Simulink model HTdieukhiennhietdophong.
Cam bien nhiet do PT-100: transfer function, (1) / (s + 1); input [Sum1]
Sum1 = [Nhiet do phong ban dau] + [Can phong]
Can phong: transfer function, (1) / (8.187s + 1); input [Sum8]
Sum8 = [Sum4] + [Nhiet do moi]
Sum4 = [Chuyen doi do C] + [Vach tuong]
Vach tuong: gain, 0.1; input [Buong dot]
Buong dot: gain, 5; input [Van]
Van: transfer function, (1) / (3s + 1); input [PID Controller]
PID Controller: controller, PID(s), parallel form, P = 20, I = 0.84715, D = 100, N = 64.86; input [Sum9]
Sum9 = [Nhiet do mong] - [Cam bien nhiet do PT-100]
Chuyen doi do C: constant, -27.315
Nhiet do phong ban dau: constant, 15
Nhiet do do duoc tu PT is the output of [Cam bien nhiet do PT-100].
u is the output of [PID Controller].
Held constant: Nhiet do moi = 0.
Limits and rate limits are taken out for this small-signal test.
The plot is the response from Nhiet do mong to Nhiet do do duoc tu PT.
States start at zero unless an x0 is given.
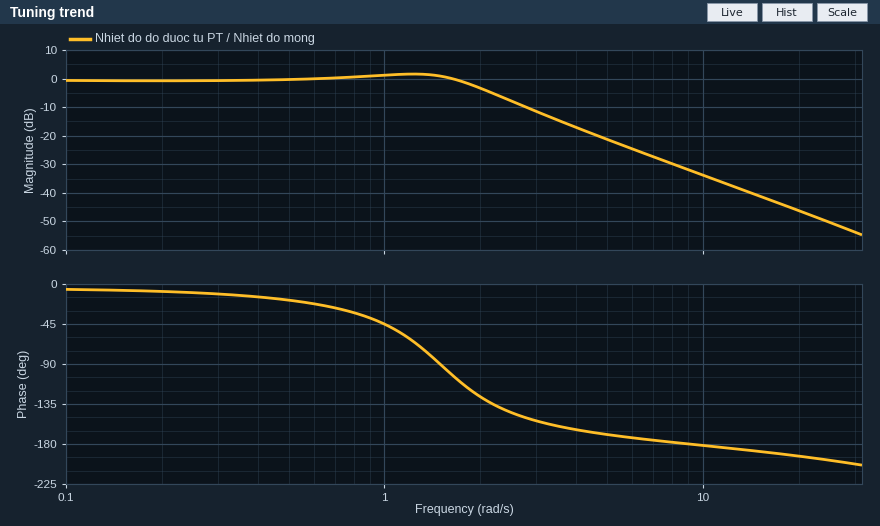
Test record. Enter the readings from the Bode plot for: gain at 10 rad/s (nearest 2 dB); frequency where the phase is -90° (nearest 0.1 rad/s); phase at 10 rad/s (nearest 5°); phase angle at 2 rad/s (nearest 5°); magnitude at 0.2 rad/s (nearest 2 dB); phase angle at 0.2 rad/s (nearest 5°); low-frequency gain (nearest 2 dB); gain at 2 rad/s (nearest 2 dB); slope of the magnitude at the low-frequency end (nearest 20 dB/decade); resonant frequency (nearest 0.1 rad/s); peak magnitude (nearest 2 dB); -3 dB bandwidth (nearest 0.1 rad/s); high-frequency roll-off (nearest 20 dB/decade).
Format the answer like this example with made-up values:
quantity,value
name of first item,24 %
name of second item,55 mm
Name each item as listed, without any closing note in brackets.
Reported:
quantity,value
gain at 10 rad/s,-34 dB
frequency where the phase is -90°,1.5 rad/s
phase at 10 rad/s,-180°
phase angle at 2 rad/s,-125°
magnitude at 0.2 rad/s,0 dB
phase angle at 0.2 rad/s,-10°
low-frequency gain,0 dB
gain at 2 rad/s,-4 dB
slope of the magnitude at the low-frequency end,0 dB/decade
resonant frequency,1.2 rad/s
peak magnitude,2 dB
-3 dB bandwidth,2.0 rad/s
high-frequency roll-off,-40 dB/decade
